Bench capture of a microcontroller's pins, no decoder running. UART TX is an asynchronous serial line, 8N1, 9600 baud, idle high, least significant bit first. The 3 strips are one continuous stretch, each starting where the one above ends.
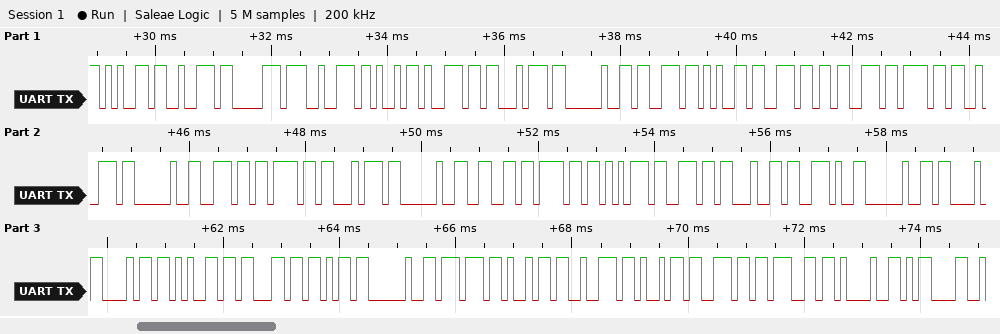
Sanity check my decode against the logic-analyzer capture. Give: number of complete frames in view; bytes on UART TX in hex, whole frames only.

40
0x65 0x72 0x70 0x72 0x69 0x6E 0x74 0x20 0x73 0x65 0x6E 0x73 0x6F 0x72 0x20 0x6E 0x6F 0x74 0x20 0x66 0x6F 0x75 0x6E 0x64 0x2E 0x20 0x43 0x68 0x65 0x63 0x6B 0x20 0x77 0x69 0x72 0x69 0x6E 0x67 0x21 0x0D
